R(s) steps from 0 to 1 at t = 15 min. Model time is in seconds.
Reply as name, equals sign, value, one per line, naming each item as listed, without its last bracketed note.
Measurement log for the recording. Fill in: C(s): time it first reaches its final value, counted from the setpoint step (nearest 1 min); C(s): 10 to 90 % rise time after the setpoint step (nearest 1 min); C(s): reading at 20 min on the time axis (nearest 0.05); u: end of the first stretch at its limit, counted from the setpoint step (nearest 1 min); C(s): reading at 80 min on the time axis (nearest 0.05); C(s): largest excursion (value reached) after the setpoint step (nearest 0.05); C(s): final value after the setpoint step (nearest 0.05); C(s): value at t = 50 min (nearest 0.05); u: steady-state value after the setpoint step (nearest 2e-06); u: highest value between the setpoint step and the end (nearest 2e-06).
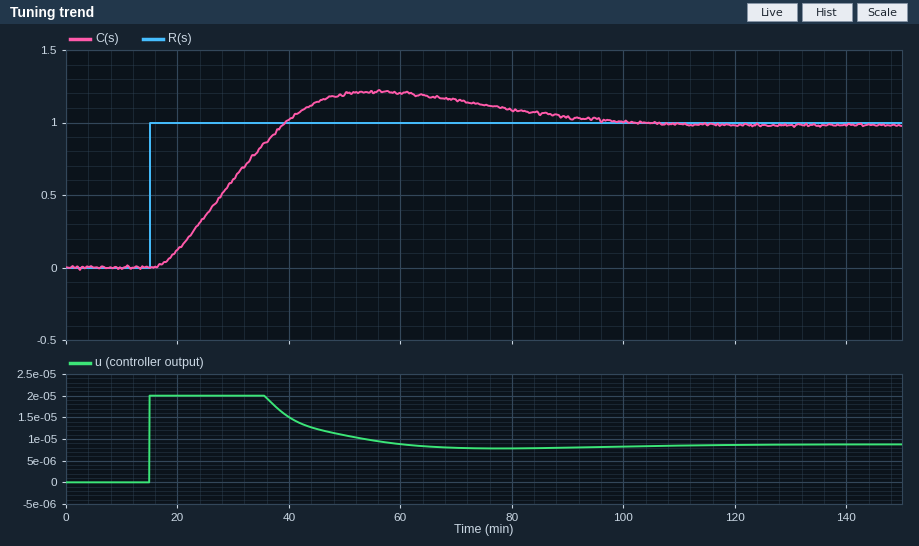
C(s): time it first reaches its final value, counted from the setpoint step = 24 min
C(s): 10 to 90 % rise time after the setpoint step = 17 min
C(s): reading at 20 min on the time axis = 0.10
u: end of the first stretch at its limit, counted from the setpoint step = 21 min
C(s): reading at 80 min on the time axis = 1.10
C(s): largest excursion (value reached) after the setpoint step = 1.20
C(s): final value after the setpoint step = 1.00
C(s): value at t = 50 min = 1.20
u: steady-state value after the setpoint step = 0.000008
u: highest value between the setpoint step and the end = 0.000020
